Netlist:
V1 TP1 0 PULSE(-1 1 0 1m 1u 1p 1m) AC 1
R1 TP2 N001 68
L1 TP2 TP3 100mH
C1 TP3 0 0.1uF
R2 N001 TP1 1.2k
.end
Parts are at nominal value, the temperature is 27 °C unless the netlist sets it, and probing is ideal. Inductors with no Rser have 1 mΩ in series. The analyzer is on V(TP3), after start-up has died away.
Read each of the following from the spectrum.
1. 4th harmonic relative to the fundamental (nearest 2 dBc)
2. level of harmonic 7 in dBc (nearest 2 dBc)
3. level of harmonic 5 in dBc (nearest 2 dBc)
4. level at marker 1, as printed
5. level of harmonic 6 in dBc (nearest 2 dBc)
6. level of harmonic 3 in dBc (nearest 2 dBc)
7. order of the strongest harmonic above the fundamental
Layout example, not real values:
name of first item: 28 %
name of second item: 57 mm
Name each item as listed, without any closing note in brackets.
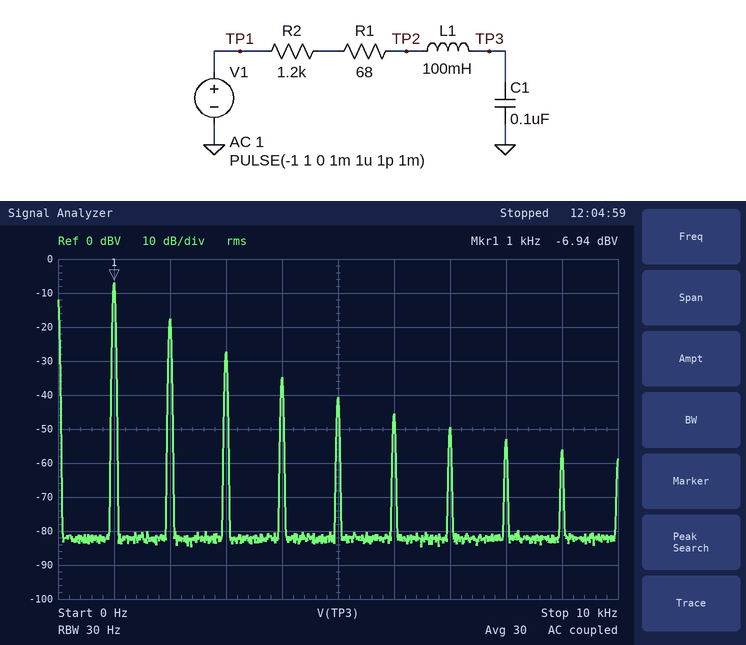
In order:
4th harmonic relative to the fundamental: -28 dBc
level of harmonic 7 in dBc: -42 dBc
level of harmonic 5 in dBc: -34 dBc
level at marker 1, as printed: -6.94 dBV
level of harmonic 6 in dBc: -38 dBc
level of harmonic 3 in dBc: -20 dBc
order of the strongest harmonic above the fundamental: 2
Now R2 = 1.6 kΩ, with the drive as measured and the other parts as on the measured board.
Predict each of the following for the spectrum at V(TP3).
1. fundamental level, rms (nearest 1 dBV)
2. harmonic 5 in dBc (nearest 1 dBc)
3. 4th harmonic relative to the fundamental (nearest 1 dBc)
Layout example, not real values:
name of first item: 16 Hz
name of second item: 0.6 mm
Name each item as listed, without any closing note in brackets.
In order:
fundamental level, rms: -9 dBV
harmonic 5 in dBc: -33 dBc
4th harmonic relative to the fundamental: -27 dBc
